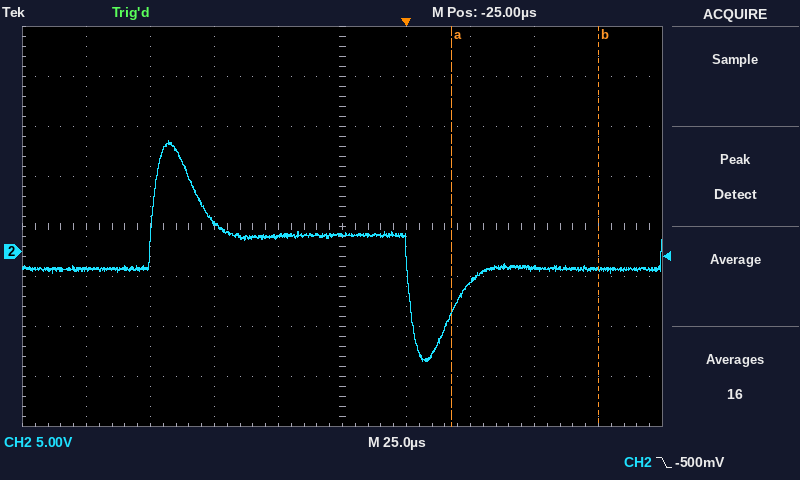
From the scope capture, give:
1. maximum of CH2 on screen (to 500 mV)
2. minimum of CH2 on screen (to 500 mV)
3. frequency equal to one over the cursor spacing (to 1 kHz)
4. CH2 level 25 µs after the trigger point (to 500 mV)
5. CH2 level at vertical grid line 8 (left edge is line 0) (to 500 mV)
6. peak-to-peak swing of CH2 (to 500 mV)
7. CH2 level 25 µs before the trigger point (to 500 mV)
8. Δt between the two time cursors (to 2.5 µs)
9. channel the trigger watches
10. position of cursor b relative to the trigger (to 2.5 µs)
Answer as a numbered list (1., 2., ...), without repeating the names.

1. 11.0 V
2. -11.0 V
3. 17 kHz
4. -3.0 V
5. -1.5 V
6. 22.0 V
7. 1.5 V
8. 57.5 µs
9. CH2
10. +75.0 µs
